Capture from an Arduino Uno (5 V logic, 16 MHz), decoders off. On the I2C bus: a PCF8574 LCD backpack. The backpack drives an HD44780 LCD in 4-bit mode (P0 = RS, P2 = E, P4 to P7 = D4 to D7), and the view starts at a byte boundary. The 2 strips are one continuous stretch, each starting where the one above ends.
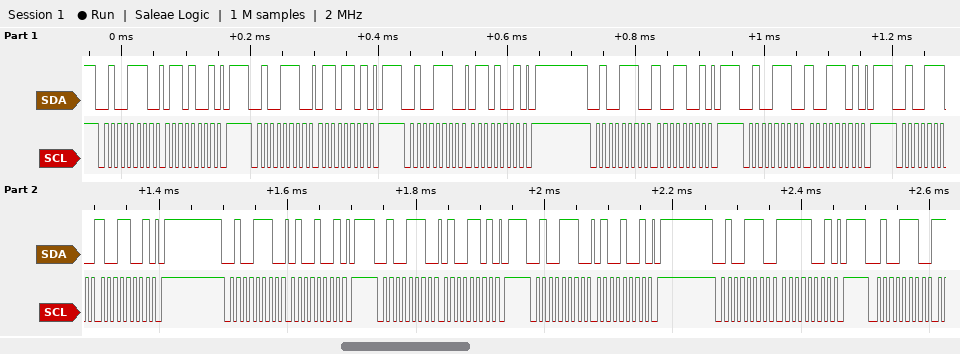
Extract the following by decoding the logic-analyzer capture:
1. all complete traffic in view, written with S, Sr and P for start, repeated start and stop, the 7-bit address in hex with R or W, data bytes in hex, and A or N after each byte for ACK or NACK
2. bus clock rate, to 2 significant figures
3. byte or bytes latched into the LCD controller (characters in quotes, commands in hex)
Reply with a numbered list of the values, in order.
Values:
1. S 27W A 69 A P S 27W A 6D A P S 27W A 69 A P S 27W A 99 A P S 27W A 9D A P S 27W A 99 A P S 27W A 49 A P S 27W A 4D A P S 27W A 49 A P S 27W A F9 A P S 27W A
2. 100 kHz
3. 'i'
